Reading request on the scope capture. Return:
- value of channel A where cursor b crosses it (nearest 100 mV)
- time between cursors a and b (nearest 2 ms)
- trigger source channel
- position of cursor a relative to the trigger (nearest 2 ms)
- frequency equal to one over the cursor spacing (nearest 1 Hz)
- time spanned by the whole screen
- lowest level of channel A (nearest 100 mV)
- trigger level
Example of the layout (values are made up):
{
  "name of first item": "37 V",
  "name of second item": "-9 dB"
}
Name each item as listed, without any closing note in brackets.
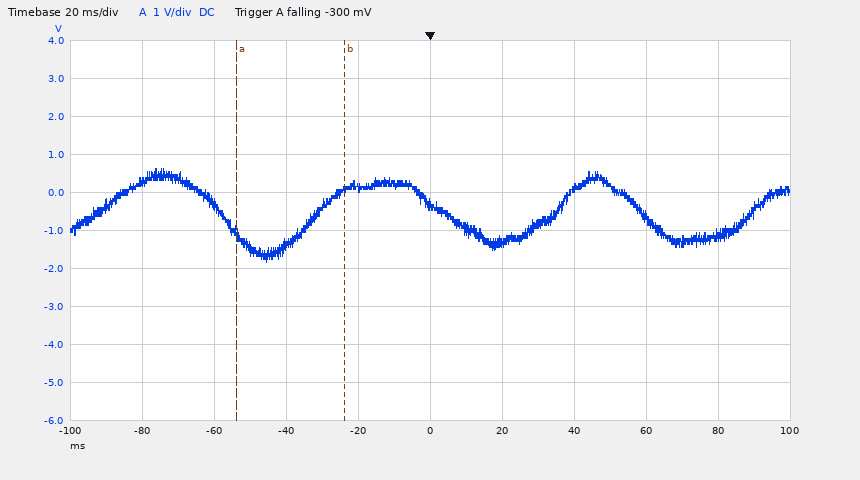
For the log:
{
  "value of channel A where cursor b crosses it": "100 mV",
  "time between cursors a and b": "30 ms",
  "trigger source channel": "channel A",
  "position of cursor a relative to the trigger": "-54 ms",
  "frequency equal to one over the cursor spacing": "33 Hz",
  "time spanned by the whole screen": "200 ms",
  "lowest level of channel A": "-1.8 V",
  "trigger level": "-300 mV"
}
